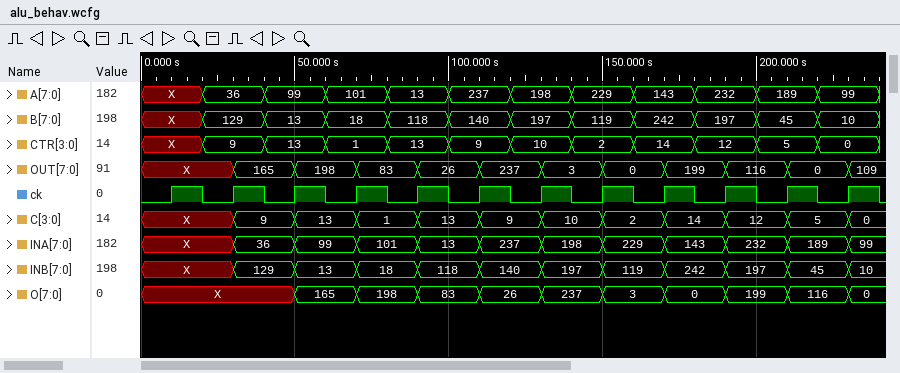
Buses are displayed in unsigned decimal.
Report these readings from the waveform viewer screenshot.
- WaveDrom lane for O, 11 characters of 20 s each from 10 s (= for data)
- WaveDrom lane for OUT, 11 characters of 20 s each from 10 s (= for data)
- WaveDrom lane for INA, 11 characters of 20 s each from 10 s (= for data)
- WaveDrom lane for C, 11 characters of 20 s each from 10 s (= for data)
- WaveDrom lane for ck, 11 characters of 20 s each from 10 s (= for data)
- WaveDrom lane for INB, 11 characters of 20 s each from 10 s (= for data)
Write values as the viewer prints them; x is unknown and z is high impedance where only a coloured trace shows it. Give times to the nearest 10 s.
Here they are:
{name: 'O', wave: 'x.=========', data: '165 198 83 26 237 3 0 199 116'}
{name: 'OUT', wave: 'x==========', data: '165 198 83 26 237 3 0 199 116 0'}
{name: 'INA', wave: 'x==========', data: '36 99 101 13 237 198 229 143 232 189'}
{name: 'C', wave: 'x==========', data: '9 13 1 13 9 10 2 14 12 5'}
{name: 'ck', wave: 'p..........'}
{name: 'INB', wave: 'x==========', data: '129 13 18 118 140 197 119 242 197 45'}
